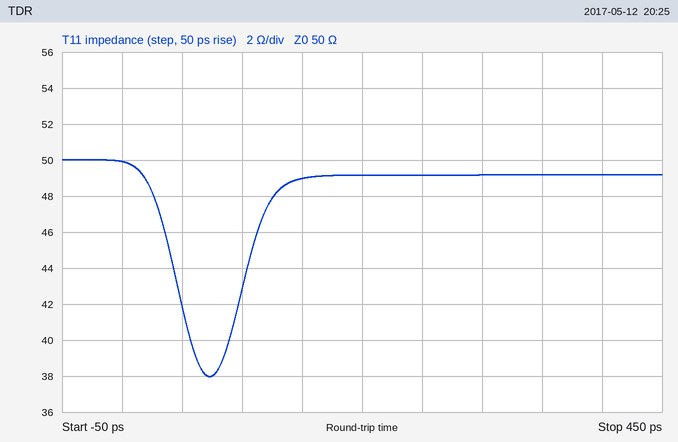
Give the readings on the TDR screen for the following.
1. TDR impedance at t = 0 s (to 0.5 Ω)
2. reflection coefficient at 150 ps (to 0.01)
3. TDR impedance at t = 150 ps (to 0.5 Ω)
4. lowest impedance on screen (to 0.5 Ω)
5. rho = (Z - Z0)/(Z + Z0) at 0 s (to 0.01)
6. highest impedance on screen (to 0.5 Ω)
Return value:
50.0 Ω
-0.01
49.0 Ω
38.0 Ω
0.00
50.0 Ω
